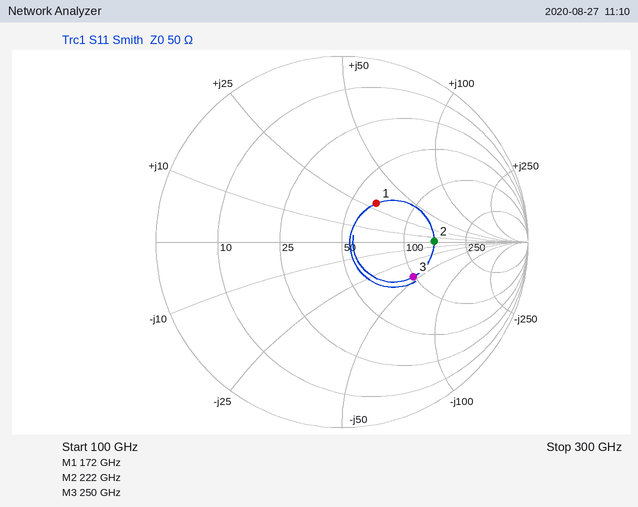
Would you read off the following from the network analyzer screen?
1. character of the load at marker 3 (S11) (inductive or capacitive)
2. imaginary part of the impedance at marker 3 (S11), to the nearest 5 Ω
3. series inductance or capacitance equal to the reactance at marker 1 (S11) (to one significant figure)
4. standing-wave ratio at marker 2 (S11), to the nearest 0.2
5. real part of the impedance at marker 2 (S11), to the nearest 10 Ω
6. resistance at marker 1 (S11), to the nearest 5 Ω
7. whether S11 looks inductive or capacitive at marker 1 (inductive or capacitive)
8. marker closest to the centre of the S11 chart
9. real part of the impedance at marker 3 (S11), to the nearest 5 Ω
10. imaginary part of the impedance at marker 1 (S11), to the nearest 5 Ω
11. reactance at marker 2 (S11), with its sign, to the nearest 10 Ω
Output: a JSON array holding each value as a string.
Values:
["capacitive", "-45 Ω", "30 pH", "3.0", "150 Ω", "65 Ω", "inductive", "marker 1", "100 Ω", "+30 Ω", "0 Ω"]
